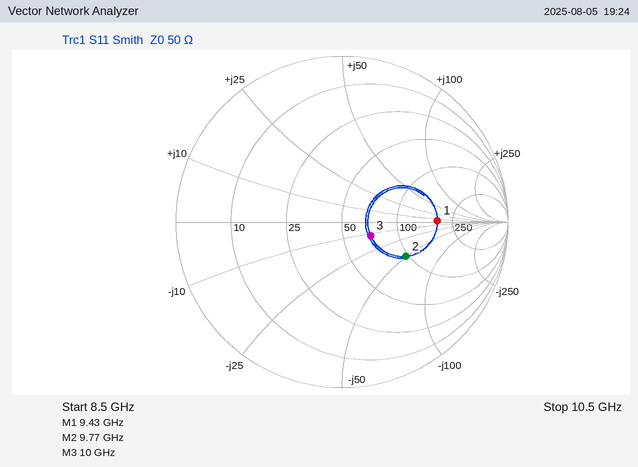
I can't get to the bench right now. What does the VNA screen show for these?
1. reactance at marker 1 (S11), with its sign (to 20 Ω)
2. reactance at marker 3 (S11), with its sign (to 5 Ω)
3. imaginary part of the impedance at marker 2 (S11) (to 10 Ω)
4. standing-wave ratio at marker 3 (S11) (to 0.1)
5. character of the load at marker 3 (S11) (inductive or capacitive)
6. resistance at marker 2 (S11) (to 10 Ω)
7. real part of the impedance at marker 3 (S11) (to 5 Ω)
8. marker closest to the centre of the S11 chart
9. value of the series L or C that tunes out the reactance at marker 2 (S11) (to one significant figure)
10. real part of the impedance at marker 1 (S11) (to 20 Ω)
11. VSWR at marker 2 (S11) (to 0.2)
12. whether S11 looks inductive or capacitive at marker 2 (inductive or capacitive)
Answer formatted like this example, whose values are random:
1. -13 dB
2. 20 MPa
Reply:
1. 0 Ω
2. -10 Ω
3. -50 Ω
4. 1.5
5. capacitive
6. 100 Ω
7. 70 Ω
8. marker 3
9. 800 pH
10. 180 Ω
11. 2.6
12. capacitive
